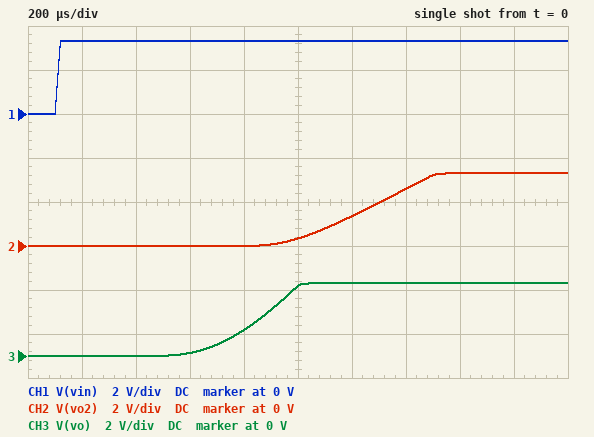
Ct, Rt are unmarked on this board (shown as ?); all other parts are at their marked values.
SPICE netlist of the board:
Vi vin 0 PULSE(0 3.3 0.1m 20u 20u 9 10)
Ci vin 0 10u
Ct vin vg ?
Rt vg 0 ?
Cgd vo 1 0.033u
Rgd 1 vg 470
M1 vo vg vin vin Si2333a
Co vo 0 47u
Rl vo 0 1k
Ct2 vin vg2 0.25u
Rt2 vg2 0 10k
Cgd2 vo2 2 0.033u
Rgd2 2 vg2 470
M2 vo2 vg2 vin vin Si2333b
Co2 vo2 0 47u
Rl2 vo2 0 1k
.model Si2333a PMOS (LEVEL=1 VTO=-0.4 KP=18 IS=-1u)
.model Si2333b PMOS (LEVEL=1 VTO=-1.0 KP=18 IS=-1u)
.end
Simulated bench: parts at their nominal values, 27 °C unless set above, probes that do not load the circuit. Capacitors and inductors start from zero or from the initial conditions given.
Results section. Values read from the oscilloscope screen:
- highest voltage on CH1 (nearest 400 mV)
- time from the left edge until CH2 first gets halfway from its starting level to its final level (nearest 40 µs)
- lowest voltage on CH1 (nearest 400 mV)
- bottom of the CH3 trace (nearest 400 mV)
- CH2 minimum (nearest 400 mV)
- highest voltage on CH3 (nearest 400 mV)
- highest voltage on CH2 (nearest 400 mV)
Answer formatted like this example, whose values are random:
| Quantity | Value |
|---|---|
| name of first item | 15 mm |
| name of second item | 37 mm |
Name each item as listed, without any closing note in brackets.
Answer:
| Quantity | Value |
|---|---|
| highest voltage on CH1 | 3.2 V |
| time from the left edge until CH2 first gets halfway from its starting level to its final level | 1.24 ms |
| lowest voltage on CH1 | 0 V |
| bottom of the CH3 trace | 0 V |
| CH2 minimum | 0 V |
| highest voltage on CH3 | 3.2 V |
| highest voltage on CH2 | 3.2 V |
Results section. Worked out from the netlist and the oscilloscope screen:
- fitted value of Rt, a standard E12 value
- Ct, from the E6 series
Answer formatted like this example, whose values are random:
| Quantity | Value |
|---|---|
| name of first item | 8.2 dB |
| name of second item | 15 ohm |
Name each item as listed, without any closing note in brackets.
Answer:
| Quantity | Value |
|---|---|
| fitted value of Rt, a standard E12 value | 5.6 kΩ |
| Ct, from the E6 series | 680 nF |
